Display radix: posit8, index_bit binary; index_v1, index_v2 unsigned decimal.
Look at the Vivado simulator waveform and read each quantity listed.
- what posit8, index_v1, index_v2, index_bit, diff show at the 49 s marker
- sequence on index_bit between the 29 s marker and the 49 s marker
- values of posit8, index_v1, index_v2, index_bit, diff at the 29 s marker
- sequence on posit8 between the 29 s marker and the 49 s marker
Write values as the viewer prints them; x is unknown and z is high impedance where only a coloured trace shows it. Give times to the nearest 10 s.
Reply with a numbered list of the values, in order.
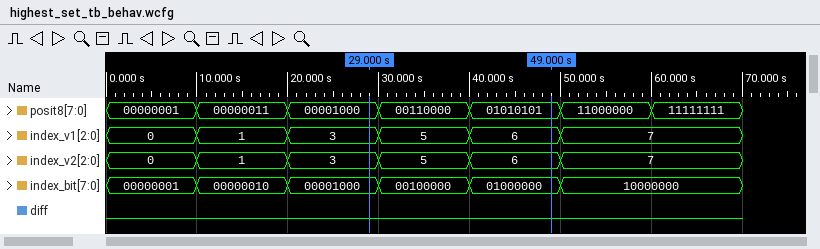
1. posit8=01010101, index_v1=6, index_v2=6, index_bit=01000000, diff=0
2. 00001000, 00100000, 01000000
3. posit8=00001000, index_v1=3, index_v2=3, index_bit=00001000, diff=0
4. 00001000, 00110000, 01010101
